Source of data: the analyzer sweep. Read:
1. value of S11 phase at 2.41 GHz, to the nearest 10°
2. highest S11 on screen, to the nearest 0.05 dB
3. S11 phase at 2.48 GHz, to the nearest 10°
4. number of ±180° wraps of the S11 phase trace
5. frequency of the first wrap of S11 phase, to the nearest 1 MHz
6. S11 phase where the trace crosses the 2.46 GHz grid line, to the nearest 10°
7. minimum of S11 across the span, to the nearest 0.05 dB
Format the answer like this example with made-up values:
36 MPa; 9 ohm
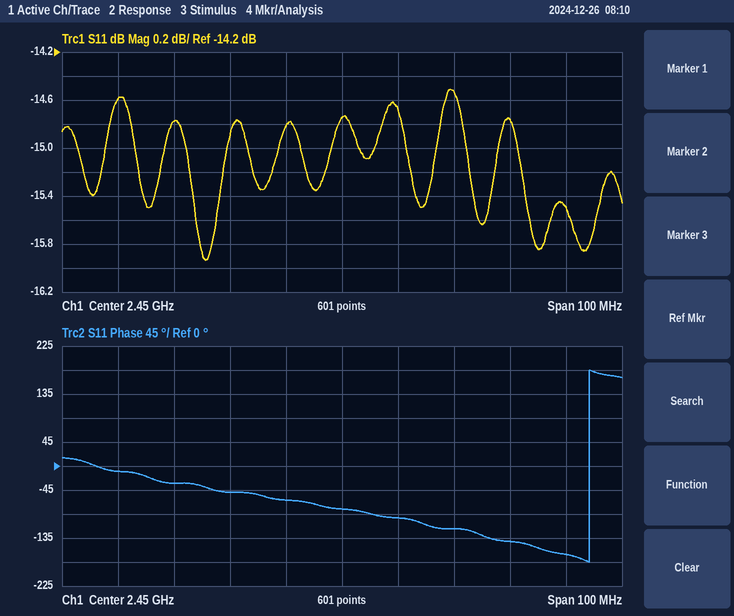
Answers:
-10°; -14.50 dB; -140°; 1; 2.494 GHz; -100°; -15.95 dB
